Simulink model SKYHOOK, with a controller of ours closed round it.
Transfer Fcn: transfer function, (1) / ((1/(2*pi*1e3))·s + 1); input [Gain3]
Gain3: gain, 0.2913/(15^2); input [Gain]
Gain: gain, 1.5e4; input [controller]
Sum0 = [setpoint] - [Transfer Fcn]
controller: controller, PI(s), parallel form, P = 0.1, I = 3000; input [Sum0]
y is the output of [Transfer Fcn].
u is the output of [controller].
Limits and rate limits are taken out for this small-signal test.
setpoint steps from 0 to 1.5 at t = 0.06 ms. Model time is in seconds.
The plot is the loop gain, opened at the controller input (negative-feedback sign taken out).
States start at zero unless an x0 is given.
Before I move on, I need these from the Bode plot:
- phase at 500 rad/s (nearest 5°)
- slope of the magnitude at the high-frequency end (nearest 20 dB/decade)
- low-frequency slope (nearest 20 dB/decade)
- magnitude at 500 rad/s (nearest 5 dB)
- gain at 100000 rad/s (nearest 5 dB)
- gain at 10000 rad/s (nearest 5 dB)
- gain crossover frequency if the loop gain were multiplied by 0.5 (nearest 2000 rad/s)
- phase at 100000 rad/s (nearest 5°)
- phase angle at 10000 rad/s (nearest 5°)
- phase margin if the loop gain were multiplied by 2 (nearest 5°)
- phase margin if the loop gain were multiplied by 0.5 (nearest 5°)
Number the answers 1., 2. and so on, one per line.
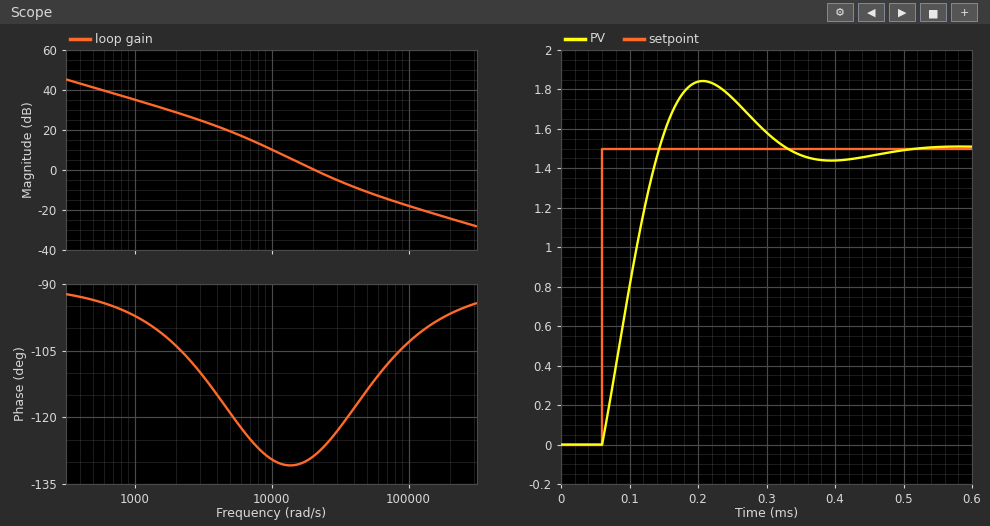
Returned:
1. -95°
2. -20 dB/decade
3. -20 dB/decade
4. 40 dB
5. -20 dB
6. 10 dB
7. 14000 rad/s
8. -105°
9. -130°
10. 60°
11. 50°
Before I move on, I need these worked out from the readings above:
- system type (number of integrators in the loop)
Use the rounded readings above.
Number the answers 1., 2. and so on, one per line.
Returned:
1. 1
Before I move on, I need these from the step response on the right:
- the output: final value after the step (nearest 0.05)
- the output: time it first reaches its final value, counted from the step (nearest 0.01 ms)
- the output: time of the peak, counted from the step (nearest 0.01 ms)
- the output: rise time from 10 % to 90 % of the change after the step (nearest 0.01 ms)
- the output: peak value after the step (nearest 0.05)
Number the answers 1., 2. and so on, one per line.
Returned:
1. 1.50
2. 0.08 ms
3. 0.15 ms
4. 0.06 ms
5. 1.85
